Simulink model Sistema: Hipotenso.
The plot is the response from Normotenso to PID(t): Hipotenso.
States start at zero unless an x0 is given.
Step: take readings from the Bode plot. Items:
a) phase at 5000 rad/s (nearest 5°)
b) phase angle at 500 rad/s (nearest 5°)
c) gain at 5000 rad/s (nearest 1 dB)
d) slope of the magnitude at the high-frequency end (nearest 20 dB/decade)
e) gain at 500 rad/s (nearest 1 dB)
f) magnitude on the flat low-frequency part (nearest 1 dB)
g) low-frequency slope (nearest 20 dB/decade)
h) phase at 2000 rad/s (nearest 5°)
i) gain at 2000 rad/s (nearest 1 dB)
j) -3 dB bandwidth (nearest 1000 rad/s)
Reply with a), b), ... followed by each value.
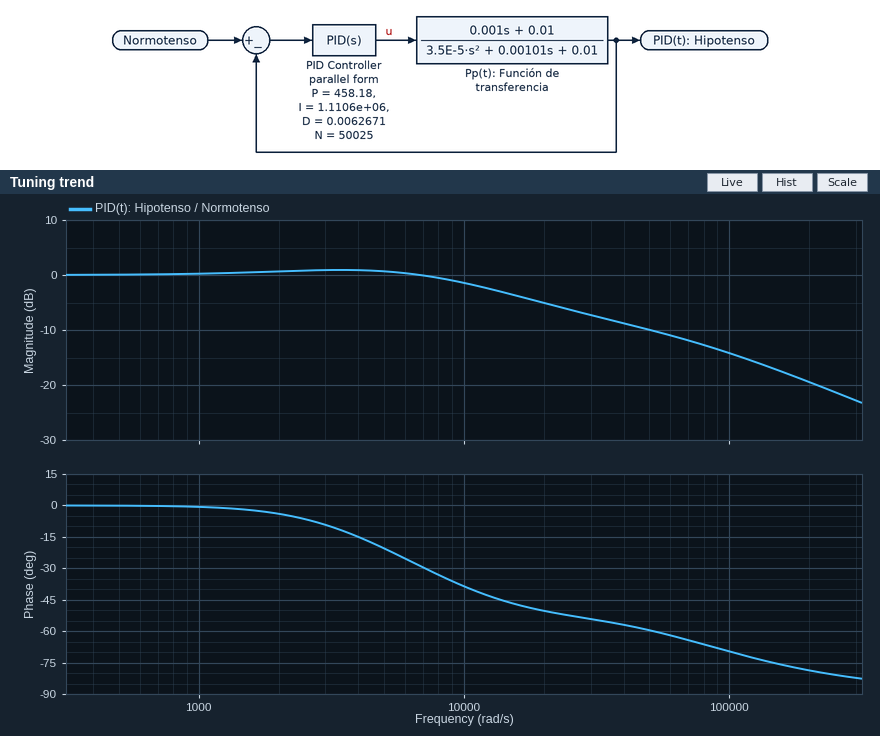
a) -20°
b) 0°
c) 1 dB
d) -20 dB/decade
e) 0 dB
f) 0 dB
g) 0 dB/decade
h) -5°
i) 1 dB
j) 14000 rad/s
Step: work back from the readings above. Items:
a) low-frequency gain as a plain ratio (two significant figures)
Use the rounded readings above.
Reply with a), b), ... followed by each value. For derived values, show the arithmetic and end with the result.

a) 10^(0 / 20) = 1.0
